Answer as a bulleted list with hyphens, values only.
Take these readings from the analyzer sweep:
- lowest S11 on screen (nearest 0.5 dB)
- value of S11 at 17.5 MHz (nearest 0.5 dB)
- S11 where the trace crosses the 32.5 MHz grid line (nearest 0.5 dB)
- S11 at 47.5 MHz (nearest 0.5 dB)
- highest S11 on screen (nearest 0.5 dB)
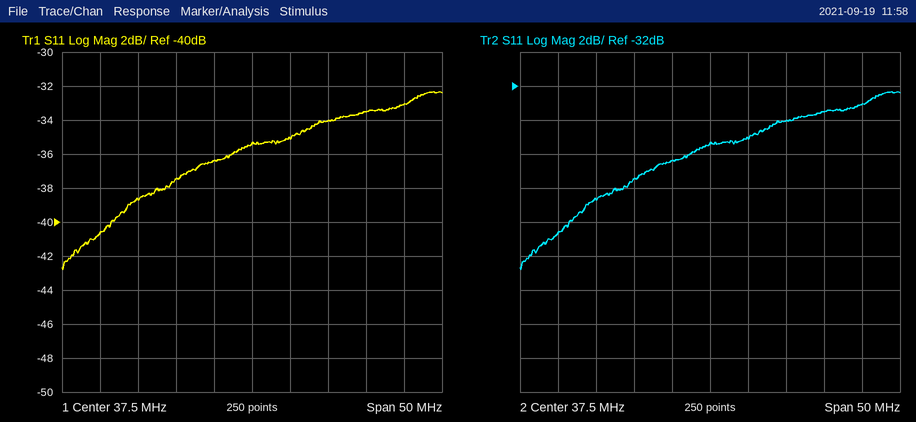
- -43.0 dB
- -40.5 dB
- -36.5 dB
- -34.0 dB
- -32.5 dB
